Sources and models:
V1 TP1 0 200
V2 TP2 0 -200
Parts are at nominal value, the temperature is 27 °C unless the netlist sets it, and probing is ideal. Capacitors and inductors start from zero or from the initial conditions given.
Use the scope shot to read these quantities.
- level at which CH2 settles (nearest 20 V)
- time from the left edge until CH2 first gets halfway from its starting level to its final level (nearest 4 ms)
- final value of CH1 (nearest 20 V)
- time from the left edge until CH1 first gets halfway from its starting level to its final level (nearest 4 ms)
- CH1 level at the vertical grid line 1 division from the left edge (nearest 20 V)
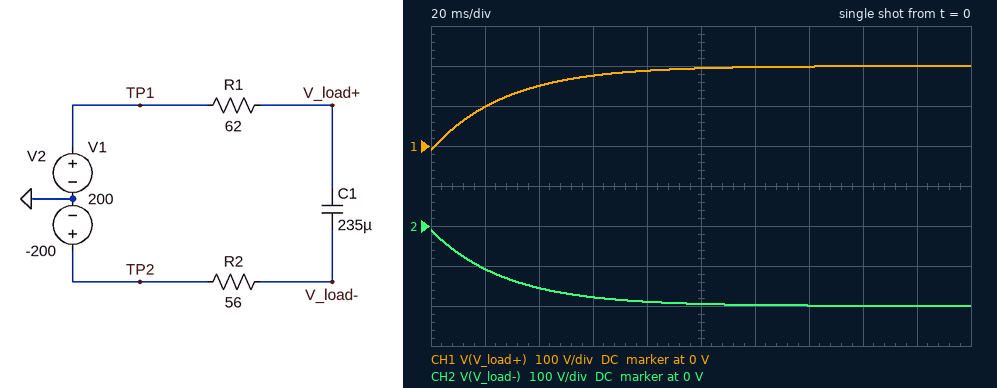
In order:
-200 V
20 ms
200 V
20 ms
100 V
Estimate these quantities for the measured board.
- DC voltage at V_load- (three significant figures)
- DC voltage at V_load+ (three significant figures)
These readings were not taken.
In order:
-200 V
200 V
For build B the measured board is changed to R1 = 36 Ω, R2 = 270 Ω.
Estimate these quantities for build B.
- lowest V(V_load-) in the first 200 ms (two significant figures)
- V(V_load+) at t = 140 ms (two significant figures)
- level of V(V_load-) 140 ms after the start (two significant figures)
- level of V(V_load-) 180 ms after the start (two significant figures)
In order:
-180 V
190 V
-150 V
-170 V
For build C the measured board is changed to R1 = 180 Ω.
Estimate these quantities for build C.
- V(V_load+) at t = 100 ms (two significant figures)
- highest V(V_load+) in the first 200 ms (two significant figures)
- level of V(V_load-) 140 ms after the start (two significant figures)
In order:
150 V
190 V
-190 V
